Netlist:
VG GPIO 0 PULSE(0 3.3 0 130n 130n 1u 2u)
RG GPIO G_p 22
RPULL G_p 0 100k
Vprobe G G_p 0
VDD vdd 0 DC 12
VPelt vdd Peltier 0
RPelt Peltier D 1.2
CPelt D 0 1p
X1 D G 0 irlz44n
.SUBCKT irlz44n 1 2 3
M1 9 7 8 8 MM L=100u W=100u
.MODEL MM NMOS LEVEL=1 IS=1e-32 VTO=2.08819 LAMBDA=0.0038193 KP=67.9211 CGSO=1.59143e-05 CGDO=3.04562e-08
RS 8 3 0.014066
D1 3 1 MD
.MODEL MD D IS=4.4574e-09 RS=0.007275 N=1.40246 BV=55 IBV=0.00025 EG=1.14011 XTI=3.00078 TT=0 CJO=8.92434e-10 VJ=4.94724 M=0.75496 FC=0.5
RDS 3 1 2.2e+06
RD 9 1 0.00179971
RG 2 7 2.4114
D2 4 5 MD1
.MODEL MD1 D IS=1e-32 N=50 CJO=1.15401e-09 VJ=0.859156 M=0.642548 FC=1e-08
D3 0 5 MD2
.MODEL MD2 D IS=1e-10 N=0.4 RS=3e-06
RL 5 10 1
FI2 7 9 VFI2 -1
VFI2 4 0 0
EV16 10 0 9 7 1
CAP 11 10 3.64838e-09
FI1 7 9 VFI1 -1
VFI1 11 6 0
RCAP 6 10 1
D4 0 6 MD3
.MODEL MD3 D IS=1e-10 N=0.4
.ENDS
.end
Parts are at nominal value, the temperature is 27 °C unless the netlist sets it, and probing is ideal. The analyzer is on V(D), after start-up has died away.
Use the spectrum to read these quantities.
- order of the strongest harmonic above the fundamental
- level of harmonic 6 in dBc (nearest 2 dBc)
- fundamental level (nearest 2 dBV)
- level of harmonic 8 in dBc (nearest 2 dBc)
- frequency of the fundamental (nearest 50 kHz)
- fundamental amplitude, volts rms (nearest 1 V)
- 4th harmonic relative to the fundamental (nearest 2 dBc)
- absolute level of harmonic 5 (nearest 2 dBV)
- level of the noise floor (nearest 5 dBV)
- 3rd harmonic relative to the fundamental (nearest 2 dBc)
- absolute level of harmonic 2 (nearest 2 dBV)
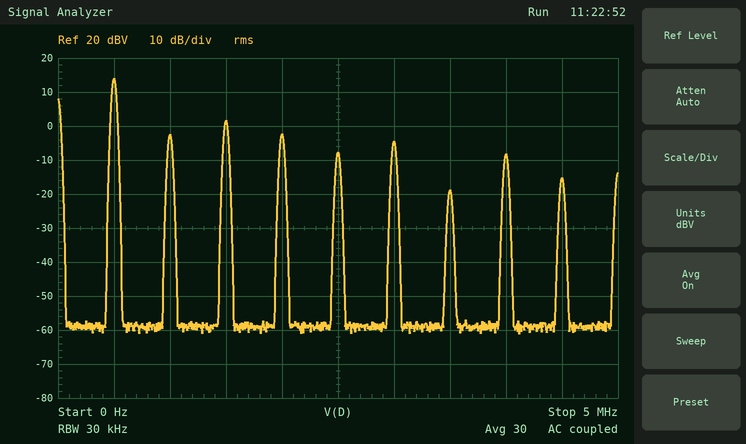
3
-18 dBc
14 dBV
-22 dBc
500 kHz
5 V
-16 dBc
-8 dBV
-60 dBV
-12 dBc
-2 dBV
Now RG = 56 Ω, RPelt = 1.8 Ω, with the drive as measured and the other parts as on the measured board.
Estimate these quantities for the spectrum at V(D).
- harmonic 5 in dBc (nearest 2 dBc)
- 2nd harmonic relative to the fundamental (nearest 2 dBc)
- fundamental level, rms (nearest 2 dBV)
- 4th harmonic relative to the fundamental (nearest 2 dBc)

-28 dBc
-14 dBc
14 dBV
-18 dBc
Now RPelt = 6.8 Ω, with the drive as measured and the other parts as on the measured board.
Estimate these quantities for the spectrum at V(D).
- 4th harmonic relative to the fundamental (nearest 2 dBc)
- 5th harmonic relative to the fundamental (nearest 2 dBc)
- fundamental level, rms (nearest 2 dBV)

-14 dBc
-28 dBc
14 dBV
